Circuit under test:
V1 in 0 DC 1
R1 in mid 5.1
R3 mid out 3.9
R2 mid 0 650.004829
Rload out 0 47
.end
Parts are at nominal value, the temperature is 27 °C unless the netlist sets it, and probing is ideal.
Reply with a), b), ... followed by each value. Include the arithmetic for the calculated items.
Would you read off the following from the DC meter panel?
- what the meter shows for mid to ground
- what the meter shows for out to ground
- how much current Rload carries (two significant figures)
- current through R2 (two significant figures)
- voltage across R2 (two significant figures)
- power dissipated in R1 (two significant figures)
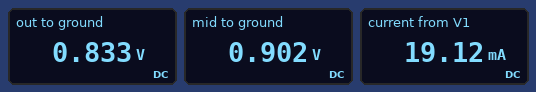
a) 0.902 V
b) 0.833 V
c) (833 mV) / 47 Ω = 18 mA
d) (902 mV) / 650 Ω = 1.4 mA
e) 902 mV = 900 mV
f) (1 V - 902 mV)^2 / 5.1 Ω = 1.9 mW
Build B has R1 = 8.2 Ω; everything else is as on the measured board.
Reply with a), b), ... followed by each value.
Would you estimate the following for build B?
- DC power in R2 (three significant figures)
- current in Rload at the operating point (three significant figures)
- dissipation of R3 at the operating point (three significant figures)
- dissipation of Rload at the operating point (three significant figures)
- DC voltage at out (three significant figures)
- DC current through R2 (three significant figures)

a) 1.12 mW
b) 16.7 mA
c) 1.09 mW
d) 13.2 mW
e) 787 mV
f) 1.31 mA
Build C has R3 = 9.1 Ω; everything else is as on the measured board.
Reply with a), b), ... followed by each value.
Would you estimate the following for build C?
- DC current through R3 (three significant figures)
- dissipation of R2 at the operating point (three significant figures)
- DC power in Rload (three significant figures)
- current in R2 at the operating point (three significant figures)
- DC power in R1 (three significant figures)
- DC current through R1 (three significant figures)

a) 16.2 mA
b) 1.27 mW
c) 12.4 mW
d) 1.40 mA
e) 1.58 mW
f) 17.6 mA
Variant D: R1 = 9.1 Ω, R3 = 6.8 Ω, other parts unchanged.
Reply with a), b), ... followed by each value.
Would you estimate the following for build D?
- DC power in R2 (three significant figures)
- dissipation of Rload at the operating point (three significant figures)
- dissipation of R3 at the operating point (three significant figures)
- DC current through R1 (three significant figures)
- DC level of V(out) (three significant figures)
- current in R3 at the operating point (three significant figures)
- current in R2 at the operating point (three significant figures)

a) 1.10 mW
b) 11.6 mW
c) 1.68 mW
d) 17.0 mA
e) 738 mV
f) 15.7 mA
g) 1.30 mA
